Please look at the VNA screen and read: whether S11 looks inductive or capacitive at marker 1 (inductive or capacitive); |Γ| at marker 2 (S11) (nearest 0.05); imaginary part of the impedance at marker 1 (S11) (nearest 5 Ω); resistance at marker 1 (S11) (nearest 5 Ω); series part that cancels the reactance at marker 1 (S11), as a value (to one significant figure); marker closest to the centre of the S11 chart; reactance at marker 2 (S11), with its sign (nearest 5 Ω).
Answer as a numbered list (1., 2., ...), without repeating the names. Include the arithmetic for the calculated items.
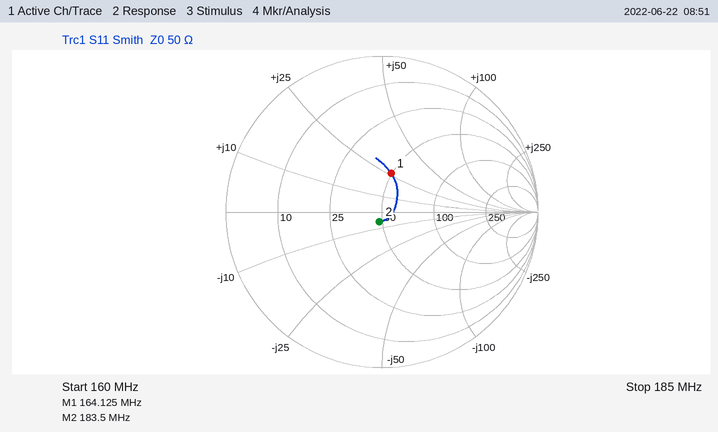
1. inductive
2. 0.05
3. +25 Ω
4. 50 Ω
5. C = 1/(2π × 164.125 MHz × 25 Ω) ≈ 38.8 pF, so 40 pF to one significant figure
6. marker 2
7. -5 Ω
